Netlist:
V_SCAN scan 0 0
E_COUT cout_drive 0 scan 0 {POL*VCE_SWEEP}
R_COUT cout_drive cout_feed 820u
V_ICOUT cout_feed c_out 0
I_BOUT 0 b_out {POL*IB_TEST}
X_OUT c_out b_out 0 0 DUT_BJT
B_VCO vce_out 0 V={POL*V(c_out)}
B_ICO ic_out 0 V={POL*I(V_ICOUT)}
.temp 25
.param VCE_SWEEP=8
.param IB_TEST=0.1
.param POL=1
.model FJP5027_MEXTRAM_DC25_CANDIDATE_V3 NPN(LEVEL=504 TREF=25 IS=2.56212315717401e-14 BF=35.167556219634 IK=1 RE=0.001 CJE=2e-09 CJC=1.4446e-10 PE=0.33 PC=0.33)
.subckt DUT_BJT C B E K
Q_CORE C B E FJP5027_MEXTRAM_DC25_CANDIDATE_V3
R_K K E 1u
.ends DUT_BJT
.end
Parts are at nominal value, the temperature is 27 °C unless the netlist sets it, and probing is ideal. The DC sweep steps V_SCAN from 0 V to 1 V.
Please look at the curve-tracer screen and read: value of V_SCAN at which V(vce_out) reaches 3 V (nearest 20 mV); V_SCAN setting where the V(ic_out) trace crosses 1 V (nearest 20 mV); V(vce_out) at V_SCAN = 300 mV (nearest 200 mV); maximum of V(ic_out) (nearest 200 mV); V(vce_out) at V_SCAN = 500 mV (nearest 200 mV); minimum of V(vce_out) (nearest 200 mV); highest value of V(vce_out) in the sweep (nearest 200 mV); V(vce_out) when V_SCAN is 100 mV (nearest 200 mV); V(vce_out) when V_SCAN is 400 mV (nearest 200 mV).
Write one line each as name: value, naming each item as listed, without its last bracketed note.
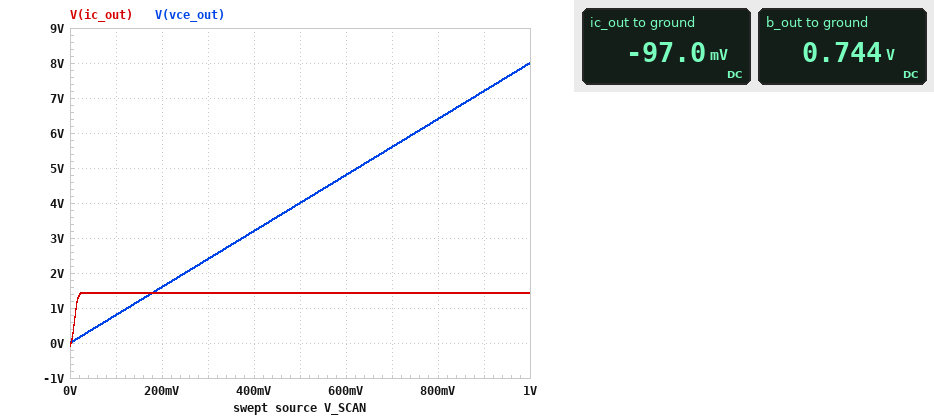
value of V_SCAN at which V(vce_out) reaches 3 V: 380 mV
V_SCAN setting where the V(ic_out) trace crosses 1 V: 20 mV
V(vce_out) at V_SCAN = 300 mV: 2.4 V
maximum of V(ic_out): 1.4 V
V(vce_out) at V_SCAN = 500 mV: 4.0 V
minimum of V(vce_out): 0 V
highest value of V(vce_out) in the sweep: 8.0 V
V(vce_out) when V_SCAN is 100 mV: 800 mV
V(vce_out) when V_SCAN is 400 mV: 3.2 V
